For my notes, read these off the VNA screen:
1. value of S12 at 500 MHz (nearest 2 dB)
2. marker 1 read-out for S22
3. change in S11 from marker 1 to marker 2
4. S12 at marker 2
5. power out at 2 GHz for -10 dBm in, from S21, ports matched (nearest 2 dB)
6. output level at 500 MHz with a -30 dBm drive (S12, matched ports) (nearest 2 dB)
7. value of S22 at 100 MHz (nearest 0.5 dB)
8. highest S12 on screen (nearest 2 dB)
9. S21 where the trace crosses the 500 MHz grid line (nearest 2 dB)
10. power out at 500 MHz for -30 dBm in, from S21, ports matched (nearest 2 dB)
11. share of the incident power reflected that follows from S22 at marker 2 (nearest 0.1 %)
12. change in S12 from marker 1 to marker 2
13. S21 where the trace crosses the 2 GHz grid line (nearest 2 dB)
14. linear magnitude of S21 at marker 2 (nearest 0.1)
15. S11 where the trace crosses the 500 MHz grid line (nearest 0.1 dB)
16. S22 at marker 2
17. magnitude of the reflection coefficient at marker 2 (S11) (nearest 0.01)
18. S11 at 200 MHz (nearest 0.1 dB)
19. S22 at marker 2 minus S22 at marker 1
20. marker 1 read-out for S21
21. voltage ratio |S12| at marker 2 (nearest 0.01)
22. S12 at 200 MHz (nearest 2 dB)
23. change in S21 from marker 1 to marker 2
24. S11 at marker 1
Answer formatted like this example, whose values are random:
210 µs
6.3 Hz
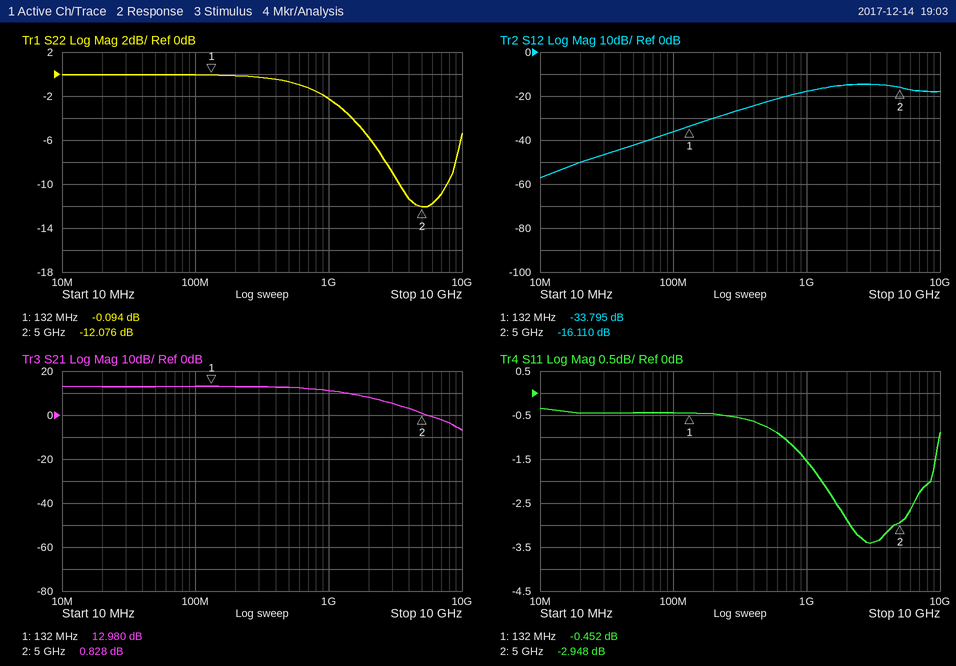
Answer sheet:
-22 dB
-0.094 dB
-2.496 dB
-16.110 dB
-2 dBm
-52 dBm
0.0 dB
-14 dB
12 dB
-18 dBm
6.2 %
17.685 dB
8 dB
1.1
-0.8 dB
-12.076 dB
0.71
-0.5 dB
-11.982 dB
12.980 dB
0.16
-30 dB
-12.152 dB
-0.452 dB
